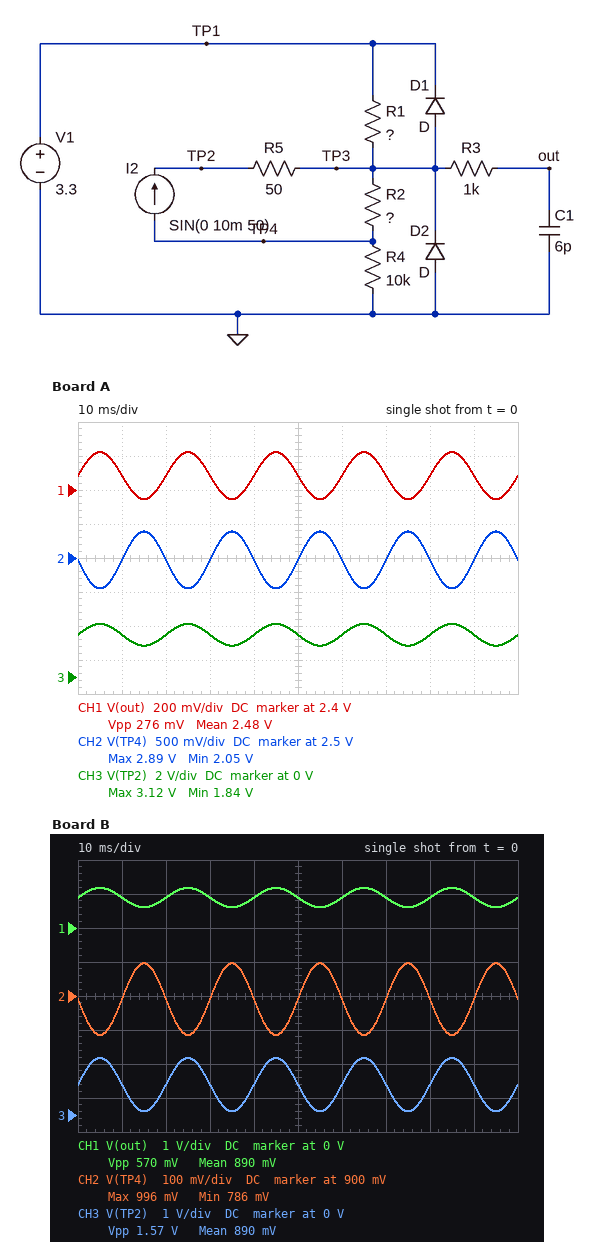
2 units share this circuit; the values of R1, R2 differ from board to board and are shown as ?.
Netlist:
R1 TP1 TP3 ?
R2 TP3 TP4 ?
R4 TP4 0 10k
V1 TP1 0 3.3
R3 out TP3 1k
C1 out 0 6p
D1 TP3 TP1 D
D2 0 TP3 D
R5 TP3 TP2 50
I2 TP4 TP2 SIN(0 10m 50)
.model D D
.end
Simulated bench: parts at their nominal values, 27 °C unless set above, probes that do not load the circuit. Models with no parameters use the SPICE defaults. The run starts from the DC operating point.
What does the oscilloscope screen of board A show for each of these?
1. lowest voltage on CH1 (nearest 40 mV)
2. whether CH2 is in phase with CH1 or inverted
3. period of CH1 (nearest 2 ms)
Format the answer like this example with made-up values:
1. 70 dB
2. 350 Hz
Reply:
1. 2.36 V
2. inverted
3. 20 ms
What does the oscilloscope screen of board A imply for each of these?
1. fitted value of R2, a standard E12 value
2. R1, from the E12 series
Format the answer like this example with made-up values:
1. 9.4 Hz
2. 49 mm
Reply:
1. 56 Ω
2. 3.3 kΩ
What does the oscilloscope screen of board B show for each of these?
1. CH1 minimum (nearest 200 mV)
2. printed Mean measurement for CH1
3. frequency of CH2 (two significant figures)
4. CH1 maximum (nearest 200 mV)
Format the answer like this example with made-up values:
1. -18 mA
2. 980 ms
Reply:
1. 600 mV
2. 890 mV
3. 50 Hz
4. 1.2 V
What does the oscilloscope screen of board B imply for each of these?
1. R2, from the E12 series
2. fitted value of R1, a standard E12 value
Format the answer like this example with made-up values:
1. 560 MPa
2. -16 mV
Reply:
1. 39 Ω
2. 27 kΩ
